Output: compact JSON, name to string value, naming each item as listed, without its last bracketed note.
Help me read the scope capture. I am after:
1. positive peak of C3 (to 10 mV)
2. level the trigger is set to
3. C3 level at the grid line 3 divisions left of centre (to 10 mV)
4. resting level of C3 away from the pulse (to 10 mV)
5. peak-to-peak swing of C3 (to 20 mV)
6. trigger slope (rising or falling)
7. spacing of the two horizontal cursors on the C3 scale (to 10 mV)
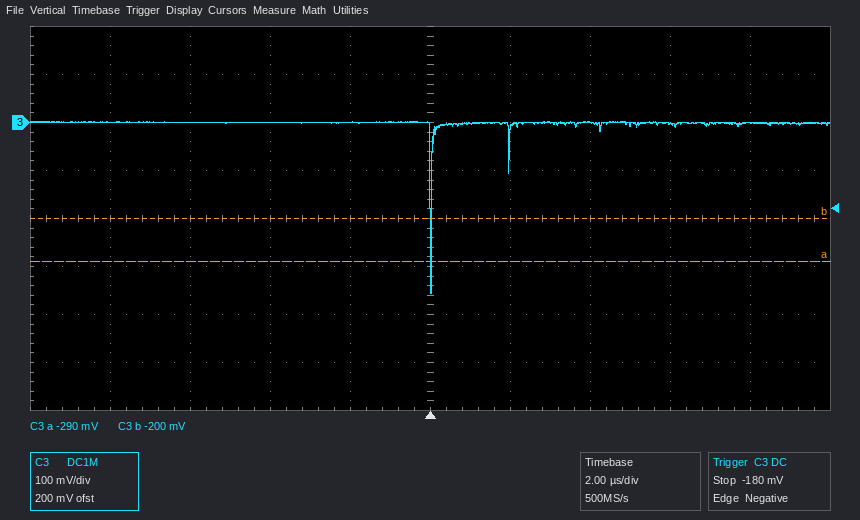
{"positive peak of C3": "0 mV", "level the trigger is set to": "-180 mV", "C3 level at the grid line 3 divisions left of centre": "0 mV", "resting level of C3 away from the pulse": "0 mV", "peak-to-peak swing of C3": "360 mV", "trigger slope": "falling", "spacing of the two horizontal cursors on the C3 scale": "90 mV"}
